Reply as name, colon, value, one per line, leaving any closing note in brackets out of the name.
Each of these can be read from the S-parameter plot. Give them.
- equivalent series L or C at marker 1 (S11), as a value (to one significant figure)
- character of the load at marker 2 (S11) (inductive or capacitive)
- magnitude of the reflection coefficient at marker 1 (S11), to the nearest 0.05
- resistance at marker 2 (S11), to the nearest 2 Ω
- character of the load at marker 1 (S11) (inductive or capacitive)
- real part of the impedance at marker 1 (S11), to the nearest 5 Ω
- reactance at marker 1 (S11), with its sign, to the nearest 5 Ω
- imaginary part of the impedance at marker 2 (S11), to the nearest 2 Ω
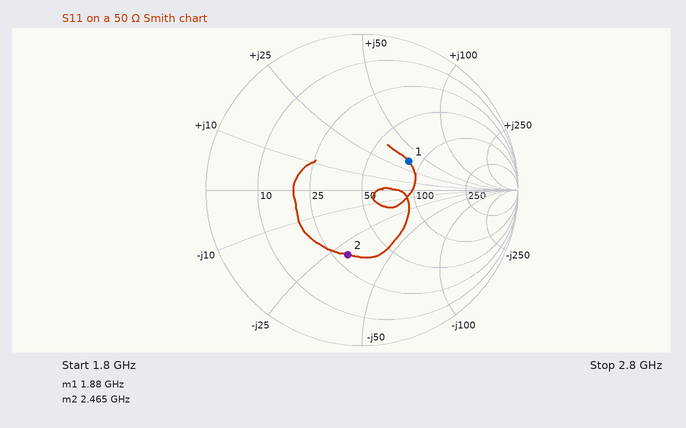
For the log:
equivalent series L or C at marker 1 (S11), as a value: 3 nH
character of the load at marker 2 (S11): capacitive
magnitude of the reflection coefficient at marker 1 (S11), to the nearest 0.05: 0.35
resistance at marker 2 (S11), to the nearest 2 Ω: 30 Ω
character of the load at marker 1 (S11): inductive
real part of the impedance at marker 1 (S11), to the nearest 5 Ω: 85 Ω
reactance at marker 1 (S11), with its sign, to the nearest 5 Ω: +35 Ω
imaginary part of the impedance at marker 2 (S11), to the nearest 2 Ω: -30 Ω
